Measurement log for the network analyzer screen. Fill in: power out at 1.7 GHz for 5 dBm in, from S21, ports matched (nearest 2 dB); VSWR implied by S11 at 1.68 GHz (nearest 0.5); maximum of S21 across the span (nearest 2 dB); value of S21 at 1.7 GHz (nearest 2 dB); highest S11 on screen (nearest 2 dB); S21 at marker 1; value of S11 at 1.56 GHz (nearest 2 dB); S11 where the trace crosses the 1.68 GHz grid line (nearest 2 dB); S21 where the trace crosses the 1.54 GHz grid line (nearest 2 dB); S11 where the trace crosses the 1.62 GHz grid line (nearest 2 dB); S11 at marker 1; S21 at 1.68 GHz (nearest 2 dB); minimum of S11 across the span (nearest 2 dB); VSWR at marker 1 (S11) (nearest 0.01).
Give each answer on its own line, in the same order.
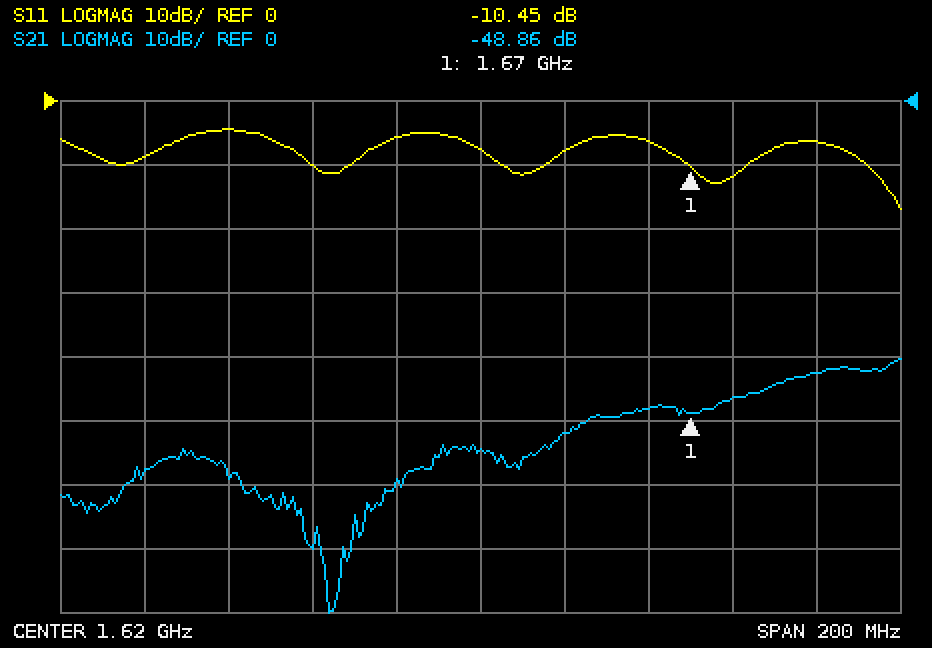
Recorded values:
-38 dBm
1.5
-40 dB
-42 dB
-4 dB
-48.86 dB
-4 dB
-12 dB
-58 dB
-8 dB
-10.45 dB
-46 dB
-16 dB
1.86
